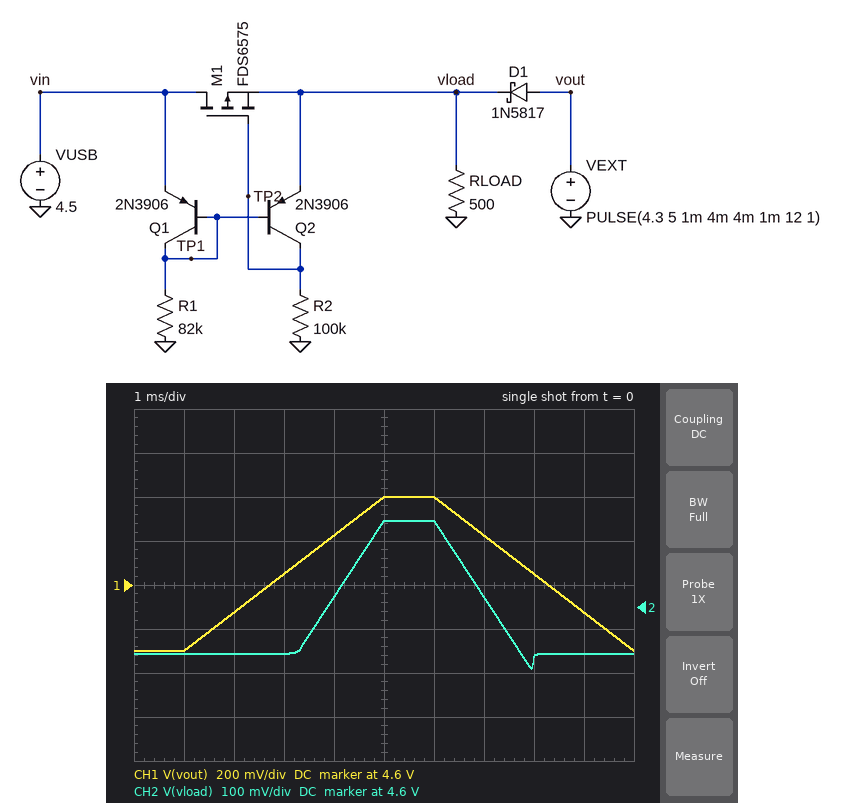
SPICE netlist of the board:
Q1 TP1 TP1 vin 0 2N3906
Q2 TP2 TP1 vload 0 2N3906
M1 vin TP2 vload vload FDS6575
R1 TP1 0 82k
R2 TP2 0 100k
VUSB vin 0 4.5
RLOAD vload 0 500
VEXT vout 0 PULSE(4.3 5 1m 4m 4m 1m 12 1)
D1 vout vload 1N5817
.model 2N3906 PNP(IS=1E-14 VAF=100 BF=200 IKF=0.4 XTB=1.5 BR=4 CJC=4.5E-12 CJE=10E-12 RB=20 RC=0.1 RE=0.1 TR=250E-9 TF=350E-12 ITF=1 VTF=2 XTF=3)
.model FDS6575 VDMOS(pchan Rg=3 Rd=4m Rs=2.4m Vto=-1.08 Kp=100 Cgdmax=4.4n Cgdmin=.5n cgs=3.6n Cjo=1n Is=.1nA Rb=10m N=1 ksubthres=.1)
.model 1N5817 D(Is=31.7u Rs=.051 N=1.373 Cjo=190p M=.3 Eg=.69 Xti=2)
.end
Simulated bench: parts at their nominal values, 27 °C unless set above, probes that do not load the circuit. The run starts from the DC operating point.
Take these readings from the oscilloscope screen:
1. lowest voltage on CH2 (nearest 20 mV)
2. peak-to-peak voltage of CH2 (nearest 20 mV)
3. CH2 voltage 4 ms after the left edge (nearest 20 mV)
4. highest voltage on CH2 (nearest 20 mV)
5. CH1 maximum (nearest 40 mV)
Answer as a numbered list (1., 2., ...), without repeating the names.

1. 4.46 V
2. 340 mV
3. 4.62 V
4. 4.80 V
5. 5.00 V
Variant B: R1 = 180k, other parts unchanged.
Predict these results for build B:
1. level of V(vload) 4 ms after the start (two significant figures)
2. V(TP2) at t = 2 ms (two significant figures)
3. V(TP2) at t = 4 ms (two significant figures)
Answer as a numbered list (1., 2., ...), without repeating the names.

1. 4.5 V
2. 2.2 V
3. 2.3 V
